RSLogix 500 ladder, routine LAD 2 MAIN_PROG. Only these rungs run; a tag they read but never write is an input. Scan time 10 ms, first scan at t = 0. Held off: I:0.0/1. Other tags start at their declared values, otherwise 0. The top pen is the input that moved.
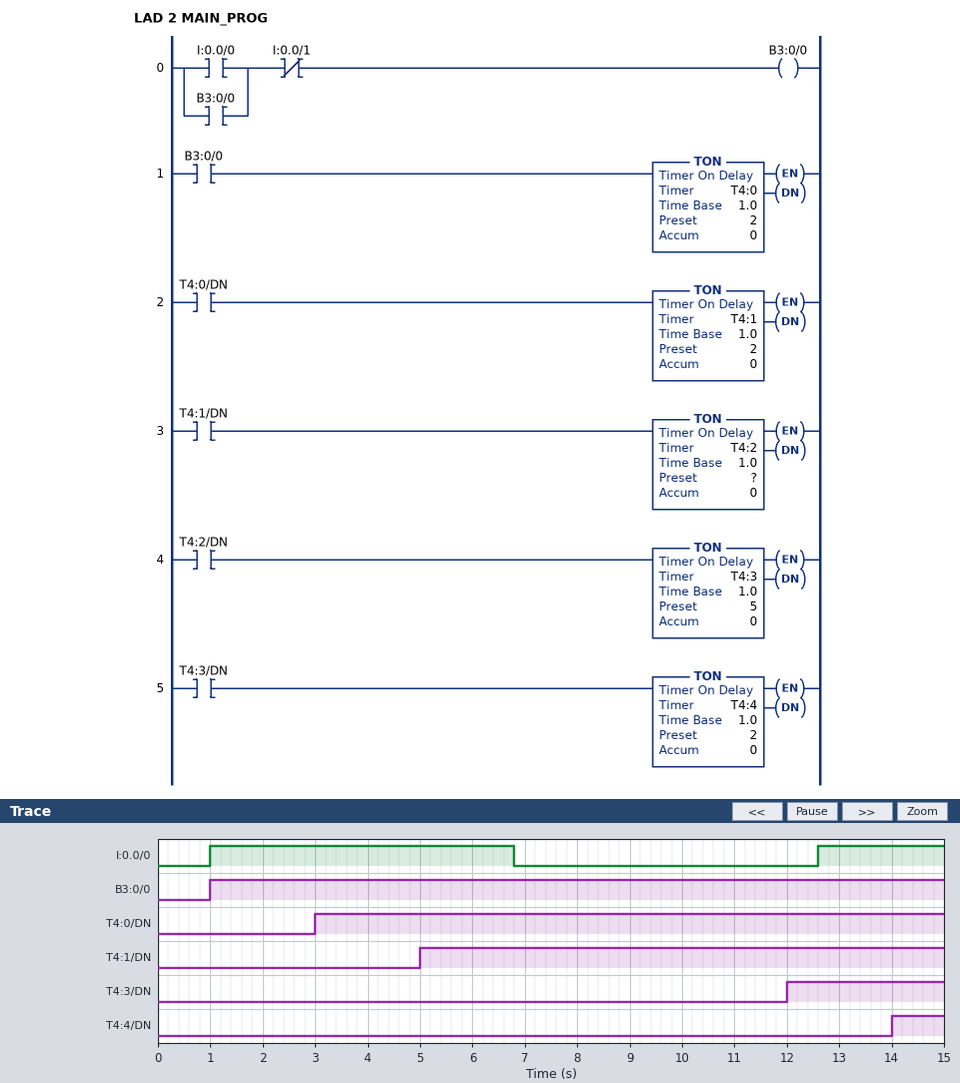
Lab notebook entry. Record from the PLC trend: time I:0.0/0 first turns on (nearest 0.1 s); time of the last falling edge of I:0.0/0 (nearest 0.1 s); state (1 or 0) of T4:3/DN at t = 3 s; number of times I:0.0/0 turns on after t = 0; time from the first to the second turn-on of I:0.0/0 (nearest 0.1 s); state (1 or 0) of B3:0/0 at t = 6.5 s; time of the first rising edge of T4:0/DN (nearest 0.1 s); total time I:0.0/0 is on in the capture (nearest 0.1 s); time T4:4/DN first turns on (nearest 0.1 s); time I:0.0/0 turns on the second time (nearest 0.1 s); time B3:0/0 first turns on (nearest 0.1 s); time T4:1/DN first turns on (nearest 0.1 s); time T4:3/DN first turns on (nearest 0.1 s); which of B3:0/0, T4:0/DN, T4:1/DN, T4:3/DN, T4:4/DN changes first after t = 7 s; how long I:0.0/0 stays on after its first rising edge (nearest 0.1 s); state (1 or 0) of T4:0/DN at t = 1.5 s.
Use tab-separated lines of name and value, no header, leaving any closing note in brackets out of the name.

time I:0.0/0 first turns on	1.0 s
time of the last falling edge of I:0.0/0	6.8 s
state (1 or 0) of T4:3/DN at t = 3 s	0
number of times I:0.0/0 turns on after t = 0	2
time from the first to the second turn-on of I:0.0/0	11.6 s
state (1 or 0) of B3:0/0 at t = 6.5 s	1
time of the first rising edge of T4:0/DN	3.0 s
total time I:0.0/0 is on in the capture	8.2 s
time T4:4/DN first turns on	14.0 s
time I:0.0/0 turns on the second time	12.6 s
time B3:0/0 first turns on	1.0 s
time T4:1/DN first turns on	5.0 s
time T4:3/DN first turns on	12.0 s
which of B3:0/0, T4:0/DN, T4:1/DN, T4:3/DN, T4:4/DN changes first after t = 7 s	T4:3/DN
how long I:0.0/0 stays on after its first rising edge	5.8 s
state (1 or 0) of T4:0/DN at t = 1.5 s	0
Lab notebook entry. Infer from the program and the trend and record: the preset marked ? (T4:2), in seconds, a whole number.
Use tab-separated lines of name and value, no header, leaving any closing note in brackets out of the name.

the preset marked ? (T4:2), in seconds, a whole number	2 s
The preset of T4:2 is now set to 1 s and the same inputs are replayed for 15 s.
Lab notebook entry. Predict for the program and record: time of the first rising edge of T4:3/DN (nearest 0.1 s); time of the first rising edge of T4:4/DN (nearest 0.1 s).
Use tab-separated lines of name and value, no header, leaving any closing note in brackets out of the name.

time of the first rising edge of T4:3/DN	11.0 s
time of the first rising edge of T4:4/DN	13.0 s
